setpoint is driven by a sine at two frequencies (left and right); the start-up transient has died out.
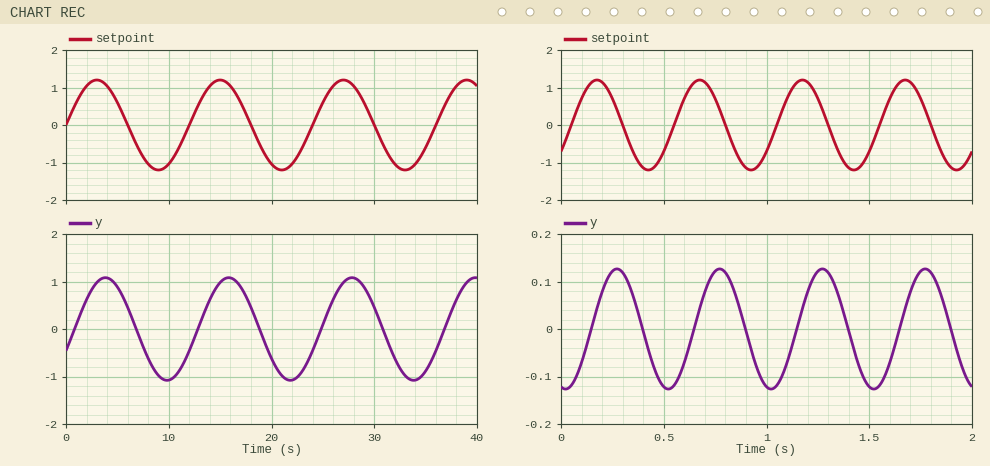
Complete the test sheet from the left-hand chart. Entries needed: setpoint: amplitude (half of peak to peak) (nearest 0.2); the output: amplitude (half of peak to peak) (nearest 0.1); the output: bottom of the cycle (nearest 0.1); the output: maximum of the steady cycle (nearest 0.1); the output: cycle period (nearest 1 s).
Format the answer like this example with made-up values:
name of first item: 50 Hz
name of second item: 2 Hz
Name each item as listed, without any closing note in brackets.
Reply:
setpoint: amplitude (half of peak to peak): 1.2
the output: amplitude (half of peak to peak): 1.1
the output: bottom of the cycle: -1.1
the output: maximum of the steady cycle: 1.1
the output: cycle period: 12 s
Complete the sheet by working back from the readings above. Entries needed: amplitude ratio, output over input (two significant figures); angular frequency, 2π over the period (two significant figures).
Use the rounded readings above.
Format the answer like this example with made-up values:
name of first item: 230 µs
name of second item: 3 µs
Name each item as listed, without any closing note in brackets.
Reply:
amplitude ratio, output over input: 0.92
angular frequency, 2π over the period: 0.52 rad/s
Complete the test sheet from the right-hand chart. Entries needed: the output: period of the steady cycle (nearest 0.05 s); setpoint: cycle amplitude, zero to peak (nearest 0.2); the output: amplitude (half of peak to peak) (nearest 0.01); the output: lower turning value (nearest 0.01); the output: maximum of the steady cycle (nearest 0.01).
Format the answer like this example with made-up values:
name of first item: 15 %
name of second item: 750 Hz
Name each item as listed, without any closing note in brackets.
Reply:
the output: period of the steady cycle: 0.50 s
setpoint: cycle amplitude, zero to peak: 1.2
the output: amplitude (half of peak to peak): 0.13
the output: lower turning value: -0.13
the output: maximum of the steady cycle: 0.13
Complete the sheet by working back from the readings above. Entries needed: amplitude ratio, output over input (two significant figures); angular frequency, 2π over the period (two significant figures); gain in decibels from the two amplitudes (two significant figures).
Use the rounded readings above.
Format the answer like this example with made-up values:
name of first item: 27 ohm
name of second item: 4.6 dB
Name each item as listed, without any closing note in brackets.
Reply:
amplitude ratio, output over input: 0.11
angular frequency, 2π over the period: 13 rad/s
gain in decibels from the two amplitudes: -19 dB
